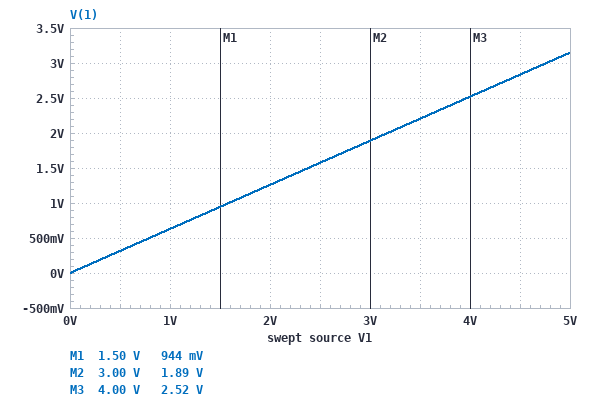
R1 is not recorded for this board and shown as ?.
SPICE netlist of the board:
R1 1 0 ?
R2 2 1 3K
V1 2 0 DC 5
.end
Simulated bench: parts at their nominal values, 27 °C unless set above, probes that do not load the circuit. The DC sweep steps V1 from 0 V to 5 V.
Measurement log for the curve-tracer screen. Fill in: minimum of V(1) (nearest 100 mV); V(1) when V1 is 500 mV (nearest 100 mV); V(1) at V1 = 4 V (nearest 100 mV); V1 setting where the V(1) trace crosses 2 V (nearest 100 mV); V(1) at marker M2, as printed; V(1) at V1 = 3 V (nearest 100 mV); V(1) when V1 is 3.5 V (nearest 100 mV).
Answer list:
0 V
300 mV
2.5 V
3.2 V
1.89 V
1.9 V
2.2 V
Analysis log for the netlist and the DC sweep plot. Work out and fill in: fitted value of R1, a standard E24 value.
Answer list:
5.1 kΩ
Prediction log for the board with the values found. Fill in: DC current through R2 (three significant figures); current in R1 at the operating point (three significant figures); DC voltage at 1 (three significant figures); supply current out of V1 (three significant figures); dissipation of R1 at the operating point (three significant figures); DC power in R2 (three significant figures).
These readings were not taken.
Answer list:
617 µA
617 µA
3.15 V
617 µA
1.94 mW
1.14 mW
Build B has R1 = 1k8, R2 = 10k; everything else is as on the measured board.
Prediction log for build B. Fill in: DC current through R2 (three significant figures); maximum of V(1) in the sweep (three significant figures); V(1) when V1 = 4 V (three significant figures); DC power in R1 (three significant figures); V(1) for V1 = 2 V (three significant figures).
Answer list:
424 µA
763 mV
610 mV
323 µW
305 mV
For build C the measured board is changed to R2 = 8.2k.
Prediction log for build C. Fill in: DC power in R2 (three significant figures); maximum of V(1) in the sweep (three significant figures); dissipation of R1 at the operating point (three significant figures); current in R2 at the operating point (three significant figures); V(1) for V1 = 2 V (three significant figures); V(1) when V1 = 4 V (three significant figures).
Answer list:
1.16 mW
1.92 V
721 µW
376 µA
767 mV
1.53 V
